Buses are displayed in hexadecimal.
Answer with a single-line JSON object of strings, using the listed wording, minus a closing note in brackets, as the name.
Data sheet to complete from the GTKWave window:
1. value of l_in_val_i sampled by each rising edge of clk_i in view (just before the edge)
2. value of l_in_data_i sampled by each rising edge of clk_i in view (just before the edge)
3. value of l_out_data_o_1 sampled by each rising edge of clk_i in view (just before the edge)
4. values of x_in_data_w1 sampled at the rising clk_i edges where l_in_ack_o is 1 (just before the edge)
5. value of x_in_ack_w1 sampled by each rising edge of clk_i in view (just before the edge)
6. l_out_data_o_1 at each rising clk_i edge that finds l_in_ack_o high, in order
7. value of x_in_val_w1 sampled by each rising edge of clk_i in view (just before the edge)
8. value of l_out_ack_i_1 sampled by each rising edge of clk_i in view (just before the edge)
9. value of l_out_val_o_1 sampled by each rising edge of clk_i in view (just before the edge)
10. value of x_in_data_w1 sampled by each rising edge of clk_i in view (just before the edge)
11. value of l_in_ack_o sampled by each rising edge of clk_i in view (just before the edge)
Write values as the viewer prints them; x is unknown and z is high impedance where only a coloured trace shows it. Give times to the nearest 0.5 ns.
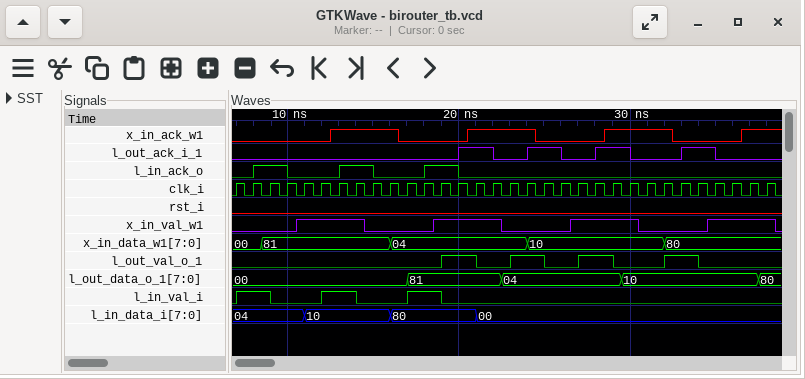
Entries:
{"value of l_in_val_i sampled by each rising edge of clk_i in view": "0 1 1 0 0 0 1 1 0 0 0 1 1 0 0 0 0 0 0 0 0 0 0 0 0 0 0 0 0 0 0 0", "value of l_in_data_i sampled by each rising edge of clk_i in view": "04, 04, 04, 04, 04, 10, 10, 10, 10, 10, 80, 80, 80, 80, 80, 00, 00, 00, 00, 00, 00, 00, 00, 00, 00, 00, 00, 00, 00, 00, 00, 00", "value of l_out_data_o_1 sampled by each rising edge of clk_i in view": "00, 00, 00, 00, 00, 00, 00, 00, 00, 00, 00, 81, 81, 81, 81, 81, 04, 04, 04, 04, 04, 04, 04, 10, 10, 10, 10, 10, 10, 10, 10, 80", "values of x_in_data_w1 sampled at the rising clk_i edges where l_in_ack_o is 1": "81, 81, 81, 81, 04, 04", "value of x_in_ack_w1 sampled by each rising edge of clk_i in view": "0 0 0 0 0 0 1 1 1 1 0 0 0 0 1 1 1 1 0 0 0 0 1 1 1 1 0 0 0 0 1 1", "l_out_data_o_1 at each rising clk_i edge that finds l_in_ack_o high, in order": "00, 00, 00, 00, 81, 81", "value of x_in_val_w1 sampled by each rising edge of clk_i in view": "0 0 0 0 1 1 1 1 0 0 0 0 1 1 1 1 0 0 0 0 1 1 1 1 0 0 0 0 1 1 1 1", "value of l_out_ack_i_1 sampled by each rising edge of clk_i in view": "0 0 0 0 0 0 0 0 0 0 0 0 0 0 1 1 0 0 1 1 0 0 1 1 0 0 0 1 1 0 0 0", "value of l_out_val_o_1 sampled by each rising edge of clk_i in view": "0 0 0 0 0 0 0 0 0 0 0 0 0 1 1 0 0 1 1 0 0 1 1 0 0 0 1 1 0 0 0 0", "value of x_in_data_w1 sampled by each rising edge of clk_i in view": "00, 00, 81, 81, 81, 81, 81, 81, 81, 81, 04, 04, 04, 04, 04, 04, 04, 04, 10, 10, 10, 10, 10, 10, 10, 10, 80, 80, 80, 80, 80, 80", "value of l_in_ack_o sampled by each rising edge of clk_i in view": "0 0 1 1 0 0 0 1 1 0 0 0 1 1 0 0 0 0 0 0 0 0 0 0 0 0 0 0 0 0 0 0"}
